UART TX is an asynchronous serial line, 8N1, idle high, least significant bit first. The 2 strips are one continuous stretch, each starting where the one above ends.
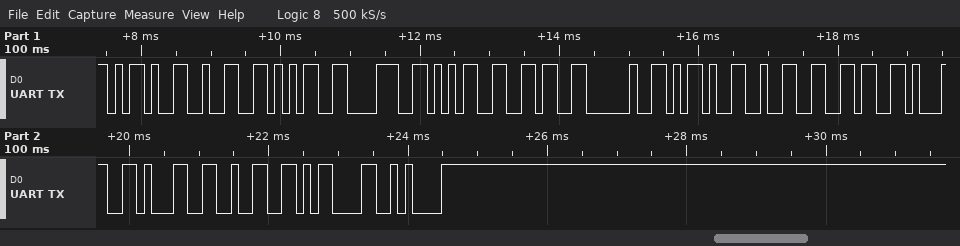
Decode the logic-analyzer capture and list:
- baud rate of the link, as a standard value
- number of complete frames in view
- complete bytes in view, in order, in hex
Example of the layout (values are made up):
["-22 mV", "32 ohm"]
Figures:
["9600 baud", "15", "2D 32 35 38 35 36 20 2D 32 36 31 31 32 0D 0A"]
